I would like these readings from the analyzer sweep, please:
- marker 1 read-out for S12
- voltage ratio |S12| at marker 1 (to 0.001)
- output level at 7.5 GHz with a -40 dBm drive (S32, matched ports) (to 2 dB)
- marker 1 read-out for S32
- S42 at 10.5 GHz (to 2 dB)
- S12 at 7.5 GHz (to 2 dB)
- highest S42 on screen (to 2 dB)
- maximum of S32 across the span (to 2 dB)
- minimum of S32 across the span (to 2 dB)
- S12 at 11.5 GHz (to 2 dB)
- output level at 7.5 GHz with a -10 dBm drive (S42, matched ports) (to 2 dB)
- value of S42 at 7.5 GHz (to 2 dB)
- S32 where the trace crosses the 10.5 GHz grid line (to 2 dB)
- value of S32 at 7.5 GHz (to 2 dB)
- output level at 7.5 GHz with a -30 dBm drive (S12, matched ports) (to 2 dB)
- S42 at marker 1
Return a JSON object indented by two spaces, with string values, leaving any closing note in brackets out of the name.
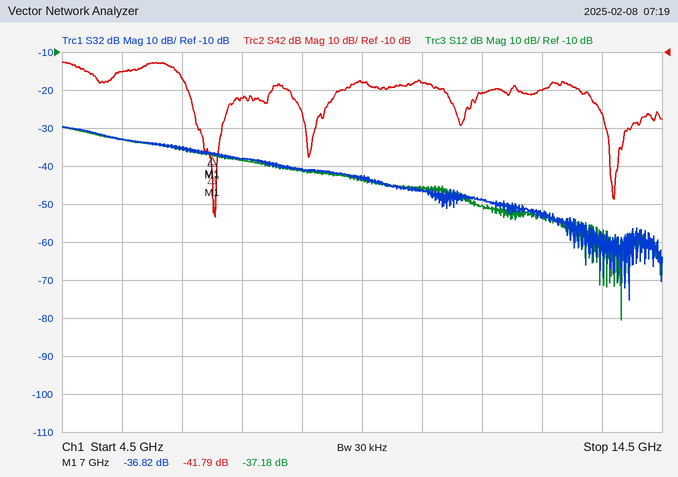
{
  "marker 1 read-out for S12": "-37.18 dB",
  "voltage ratio |S12| at marker 1": "0.014",
  "output level at 7.5 GHz with a -40 dBm drive (S32, matched ports)": "-78 dBm",
  "marker 1 read-out for S32": "-36.82 dB",
  "S42 at 10.5 GHz": "-18 dB",
  "S12 at 7.5 GHz": "-38 dB",
  "highest S42 on screen": "-12 dB",
  "maximum of S32 across the span": "-30 dB",
  "minimum of S32 across the span": "-76 dB",
  "S12 at 11.5 GHz": "-50 dB",
  "output level at 7.5 GHz with a -10 dBm drive (S42, matched ports)": "-32 dBm",
  "value of S42 at 7.5 GHz": "-22 dB",
  "S32 where the trace crosses the 10.5 GHz grid line": "-46 dB",
  "value of S32 at 7.5 GHz": "-38 dB",
  "output level at 7.5 GHz with a -30 dBm drive (S12, matched ports)": "-68 dBm",
  "S42 at marker 1": "-41.79 dB"
}
